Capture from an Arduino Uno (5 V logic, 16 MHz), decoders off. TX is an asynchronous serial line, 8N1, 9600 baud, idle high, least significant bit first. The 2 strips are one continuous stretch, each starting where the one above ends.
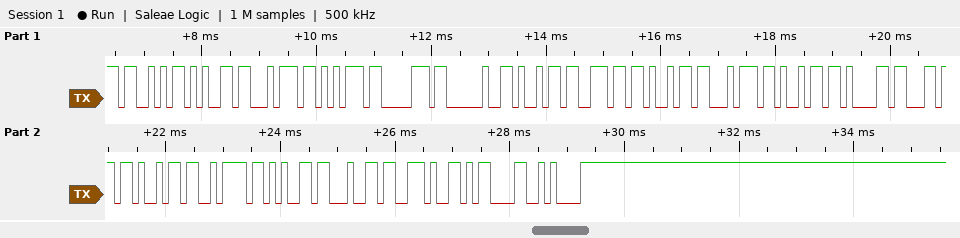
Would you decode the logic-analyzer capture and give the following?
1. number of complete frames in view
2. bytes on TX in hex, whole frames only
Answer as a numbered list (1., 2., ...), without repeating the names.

1. 20
2. 0x53 0x65 0x74 0x75 0x70 0x20 0x69 0x6E 0x69 0x74 0x69 0x61 0x6C 0x69 0x7A 0x65 0x64 0x2E 0x0D 0x0A
